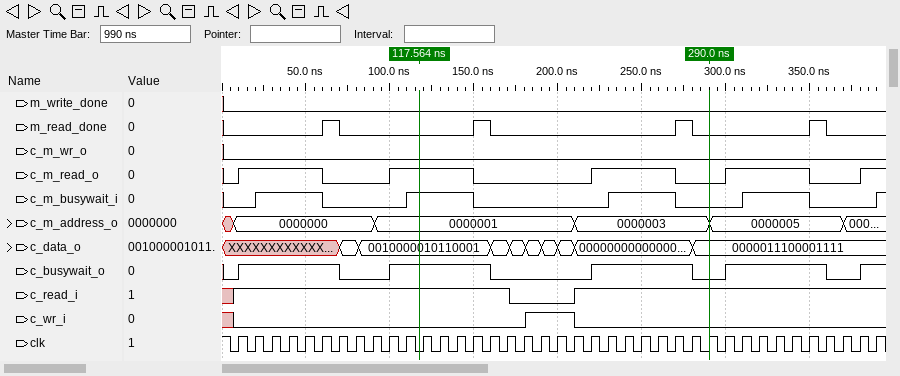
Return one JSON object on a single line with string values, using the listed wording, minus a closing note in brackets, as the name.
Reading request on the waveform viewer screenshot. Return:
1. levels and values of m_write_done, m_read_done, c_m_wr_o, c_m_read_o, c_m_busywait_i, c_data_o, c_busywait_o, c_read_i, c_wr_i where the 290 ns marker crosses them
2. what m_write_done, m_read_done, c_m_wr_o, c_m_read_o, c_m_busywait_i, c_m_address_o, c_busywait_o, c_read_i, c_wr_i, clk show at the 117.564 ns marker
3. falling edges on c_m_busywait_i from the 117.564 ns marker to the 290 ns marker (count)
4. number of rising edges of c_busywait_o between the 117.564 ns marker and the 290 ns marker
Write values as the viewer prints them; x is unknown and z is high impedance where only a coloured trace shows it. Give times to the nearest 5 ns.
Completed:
{"levels and values of m_write_done, m_read_done, c_m_wr_o, c_m_read_o, c_m_busywait_i, c_data_o, c_busywait_o, c_read_i, c_wr_i where the 290 ns marker crosses them": "m_write_done=0, m_read_done=0, c_m_wr_o=0, c_m_read_o=0, c_m_busywait_i=0, c_data_o=0000011100001111, c_busywait_o=0, c_read_i=1, c_wr_i=0", "what m_write_done, m_read_done, c_m_wr_o, c_m_read_o, c_m_busywait_i, c_m_address_o, c_busywait_o, c_read_i, c_wr_i, clk show at the 117.564 ns marker": "m_write_done=0, m_read_done=0, c_m_wr_o=0, c_m_read_o=1, c_m_busywait_i=1, c_m_address_o=0000001, c_busywait_o=1, c_read_i=1, c_wr_i=0, clk=0", "falling edges on c_m_busywait_i from the 117.564 ns marker to the 290 ns marker": "2", "number of rising edges of c_busywait_o between the 117.564 ns marker and the 290 ns marker": "1"}
